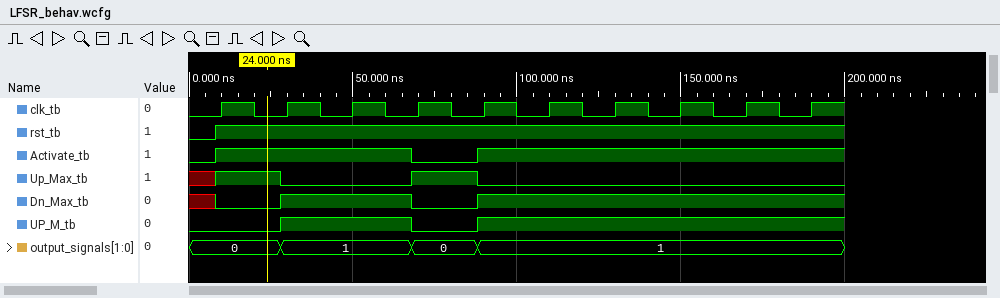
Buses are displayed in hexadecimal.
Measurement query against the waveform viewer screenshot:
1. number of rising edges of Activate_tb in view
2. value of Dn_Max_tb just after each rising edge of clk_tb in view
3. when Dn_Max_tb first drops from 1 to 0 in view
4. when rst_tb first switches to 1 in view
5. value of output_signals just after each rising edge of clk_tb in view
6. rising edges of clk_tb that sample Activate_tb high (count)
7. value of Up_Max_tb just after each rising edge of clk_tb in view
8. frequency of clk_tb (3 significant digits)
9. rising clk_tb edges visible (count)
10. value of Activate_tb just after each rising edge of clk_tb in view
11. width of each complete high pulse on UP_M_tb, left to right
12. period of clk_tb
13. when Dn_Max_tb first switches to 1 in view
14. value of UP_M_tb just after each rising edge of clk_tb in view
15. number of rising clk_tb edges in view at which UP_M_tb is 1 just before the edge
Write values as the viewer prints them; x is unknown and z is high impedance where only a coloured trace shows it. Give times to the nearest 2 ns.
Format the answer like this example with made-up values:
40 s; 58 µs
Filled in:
2; 0 1 1 0 1 1 1 1 1 1; 68 ns; 8 ns; 0, 1, 1, 0, 1, 1, 1, 1, 1, 1; 9; 1 0 0 1 0 0 0 0 0 0; 50.0 MHz; 10; 1 1 1 0 1 1 1 1 1 1; 40 ns; 20 ns; 28 ns; 0 1 1 0 1 1 1 1 1 1; 8
